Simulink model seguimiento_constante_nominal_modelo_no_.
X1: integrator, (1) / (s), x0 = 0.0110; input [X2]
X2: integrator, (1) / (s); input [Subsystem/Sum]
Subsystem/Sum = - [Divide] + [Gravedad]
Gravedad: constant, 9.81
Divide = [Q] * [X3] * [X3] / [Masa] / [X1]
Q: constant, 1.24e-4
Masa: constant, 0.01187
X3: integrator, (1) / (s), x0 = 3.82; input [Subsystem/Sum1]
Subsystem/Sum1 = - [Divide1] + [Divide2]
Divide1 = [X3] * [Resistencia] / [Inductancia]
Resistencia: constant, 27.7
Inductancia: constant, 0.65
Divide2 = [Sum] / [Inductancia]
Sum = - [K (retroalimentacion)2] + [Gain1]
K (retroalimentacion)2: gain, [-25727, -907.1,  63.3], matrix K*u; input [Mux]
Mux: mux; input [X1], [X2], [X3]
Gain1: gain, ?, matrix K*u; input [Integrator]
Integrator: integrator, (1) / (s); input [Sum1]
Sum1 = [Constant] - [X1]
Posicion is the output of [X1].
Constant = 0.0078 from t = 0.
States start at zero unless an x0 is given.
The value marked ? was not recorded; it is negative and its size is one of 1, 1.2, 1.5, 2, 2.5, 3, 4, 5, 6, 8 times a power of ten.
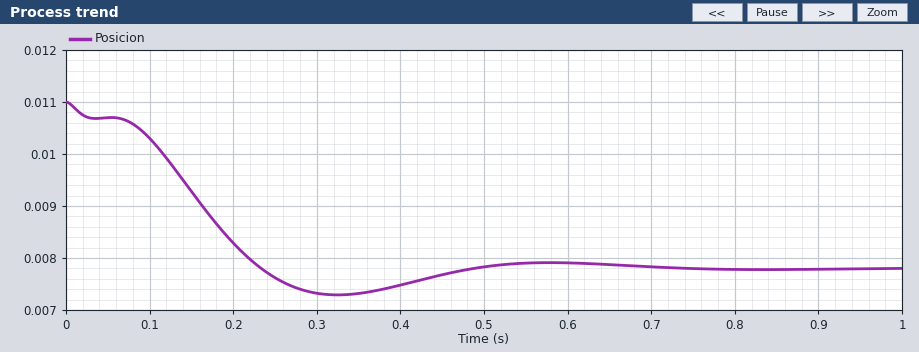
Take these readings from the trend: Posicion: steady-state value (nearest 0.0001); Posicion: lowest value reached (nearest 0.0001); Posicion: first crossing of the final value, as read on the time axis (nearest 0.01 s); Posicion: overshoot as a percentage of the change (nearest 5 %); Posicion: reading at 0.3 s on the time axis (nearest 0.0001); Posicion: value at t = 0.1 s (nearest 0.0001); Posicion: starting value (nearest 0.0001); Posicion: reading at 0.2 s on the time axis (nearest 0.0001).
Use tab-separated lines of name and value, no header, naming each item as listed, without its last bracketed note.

Posicion: steady-state value	0.0078
Posicion: lowest value reached	0.0073
Posicion: first crossing of the final value, as read on the time axis	0.23 s
Posicion: overshoot as a percentage of the change	15 %
Posicion: reading at 0.3 s on the time axis	0.0073
Posicion: value at t = 0.1 s	0.0103
Posicion: starting value	0.0110
Posicion: reading at 0.2 s on the time axis	0.0083
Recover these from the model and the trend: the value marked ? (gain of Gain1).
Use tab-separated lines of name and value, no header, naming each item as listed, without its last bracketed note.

the value marked ?	-120000
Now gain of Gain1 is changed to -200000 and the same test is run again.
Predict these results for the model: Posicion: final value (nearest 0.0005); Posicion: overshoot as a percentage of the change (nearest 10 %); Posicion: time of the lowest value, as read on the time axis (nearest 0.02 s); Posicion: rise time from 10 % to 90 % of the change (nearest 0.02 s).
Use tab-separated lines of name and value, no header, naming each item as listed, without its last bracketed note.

Posicion: final value	0.0080
Posicion: overshoot as a percentage of the change	30 %
Posicion: time of the lowest value, as read on the time axis	0.24 s
Posicion: rise time from 10 % to 90 % of the change	0.12 s
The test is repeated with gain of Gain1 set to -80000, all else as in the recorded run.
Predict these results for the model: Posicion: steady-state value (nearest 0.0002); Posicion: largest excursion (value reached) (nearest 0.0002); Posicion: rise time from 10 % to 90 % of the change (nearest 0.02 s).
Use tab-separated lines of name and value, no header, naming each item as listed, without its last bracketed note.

Posicion: steady-state value	0.0078
Posicion: largest excursion (value reached)	0.0076
Posicion: rise time from 10 % to 90 % of the change	0.20 s
